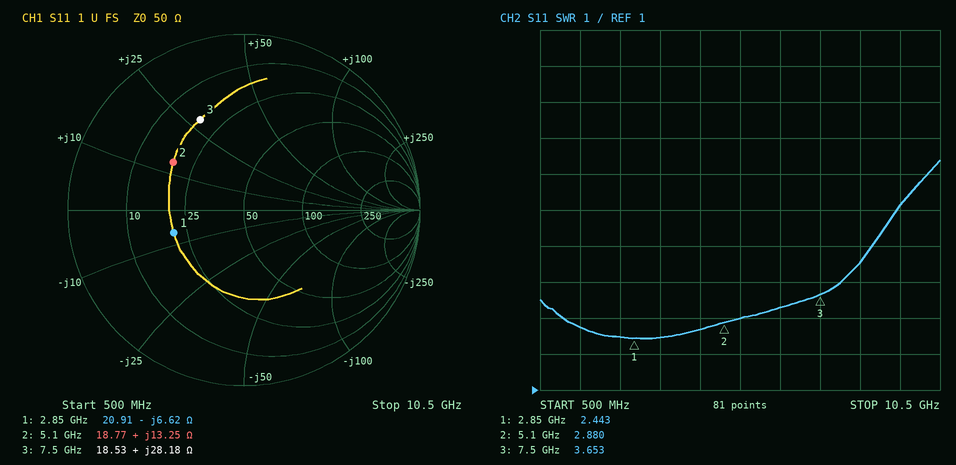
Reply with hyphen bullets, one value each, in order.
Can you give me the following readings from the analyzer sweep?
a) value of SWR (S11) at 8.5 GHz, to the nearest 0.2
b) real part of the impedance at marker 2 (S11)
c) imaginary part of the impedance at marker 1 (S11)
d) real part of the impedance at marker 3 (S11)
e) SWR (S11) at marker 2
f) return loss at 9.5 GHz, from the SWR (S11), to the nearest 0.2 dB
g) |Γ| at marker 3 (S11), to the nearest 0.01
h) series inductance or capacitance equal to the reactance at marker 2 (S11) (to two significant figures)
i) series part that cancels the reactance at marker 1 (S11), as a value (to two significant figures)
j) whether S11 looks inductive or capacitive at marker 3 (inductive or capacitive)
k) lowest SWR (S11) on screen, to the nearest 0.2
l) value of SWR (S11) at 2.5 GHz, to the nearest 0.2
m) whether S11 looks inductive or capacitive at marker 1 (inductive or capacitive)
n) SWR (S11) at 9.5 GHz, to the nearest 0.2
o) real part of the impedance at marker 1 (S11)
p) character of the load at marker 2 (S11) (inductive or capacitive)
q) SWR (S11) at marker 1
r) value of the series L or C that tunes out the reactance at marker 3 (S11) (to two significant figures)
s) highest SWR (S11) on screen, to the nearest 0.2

- 4.6
- 18.77 Ω
- -6.62 Ω
- 18.53 Ω
- 2.880
- 2.8 dB
- 0.57
- 410 pH
- 370 pH
- inductive
- 2.4
- 2.4
- capacitive
- 6.2
- 20.91 Ω
- inductive
- 2.443
- 750 fF
- 7.4
